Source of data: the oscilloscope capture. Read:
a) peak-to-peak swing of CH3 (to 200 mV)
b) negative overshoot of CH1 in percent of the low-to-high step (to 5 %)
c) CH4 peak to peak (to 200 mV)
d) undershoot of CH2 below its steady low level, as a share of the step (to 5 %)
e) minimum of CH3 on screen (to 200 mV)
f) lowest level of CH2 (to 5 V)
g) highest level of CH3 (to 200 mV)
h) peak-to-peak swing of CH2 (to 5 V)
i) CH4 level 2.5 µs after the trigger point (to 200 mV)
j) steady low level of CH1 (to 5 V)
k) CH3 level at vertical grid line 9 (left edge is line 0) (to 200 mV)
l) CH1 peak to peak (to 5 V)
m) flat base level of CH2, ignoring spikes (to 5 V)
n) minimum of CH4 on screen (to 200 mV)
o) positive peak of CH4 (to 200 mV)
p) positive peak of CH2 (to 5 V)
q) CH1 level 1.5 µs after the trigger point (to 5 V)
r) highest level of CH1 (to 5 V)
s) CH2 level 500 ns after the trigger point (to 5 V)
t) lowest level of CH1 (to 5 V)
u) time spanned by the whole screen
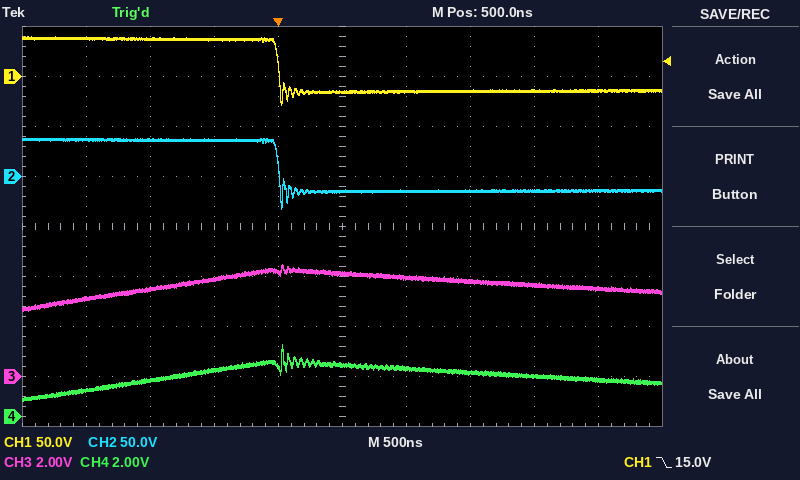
1.8 V
25 %
2.2 V
35 %
2.6 V
-30 V
4.4 V
70 V
1.4 V
-15 V
3.6 V
70 V
-15 V
600 mV
2.8 V
40 V
-15 V
40 V
-15 V
-30 V
5 µs
